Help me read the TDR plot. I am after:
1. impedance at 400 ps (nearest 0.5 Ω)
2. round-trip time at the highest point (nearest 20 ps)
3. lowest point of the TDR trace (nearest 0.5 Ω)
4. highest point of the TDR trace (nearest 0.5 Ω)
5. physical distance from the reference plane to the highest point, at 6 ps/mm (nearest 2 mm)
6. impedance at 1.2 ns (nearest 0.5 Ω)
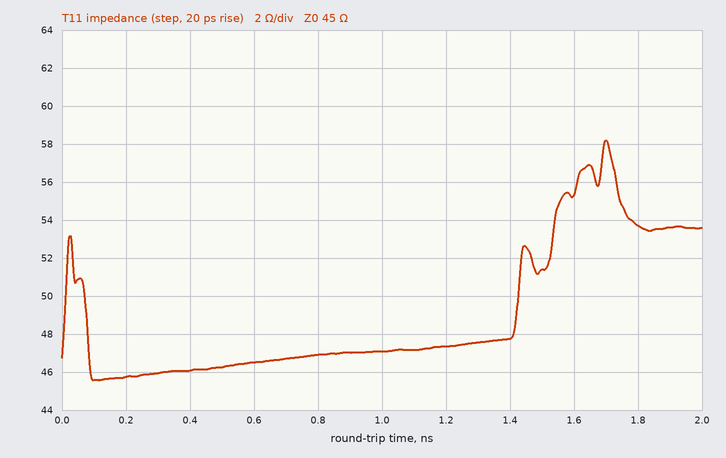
46.0 Ω
1.70 ns
45.5 Ω
58.0 Ω
142 mm
47.5 Ω
